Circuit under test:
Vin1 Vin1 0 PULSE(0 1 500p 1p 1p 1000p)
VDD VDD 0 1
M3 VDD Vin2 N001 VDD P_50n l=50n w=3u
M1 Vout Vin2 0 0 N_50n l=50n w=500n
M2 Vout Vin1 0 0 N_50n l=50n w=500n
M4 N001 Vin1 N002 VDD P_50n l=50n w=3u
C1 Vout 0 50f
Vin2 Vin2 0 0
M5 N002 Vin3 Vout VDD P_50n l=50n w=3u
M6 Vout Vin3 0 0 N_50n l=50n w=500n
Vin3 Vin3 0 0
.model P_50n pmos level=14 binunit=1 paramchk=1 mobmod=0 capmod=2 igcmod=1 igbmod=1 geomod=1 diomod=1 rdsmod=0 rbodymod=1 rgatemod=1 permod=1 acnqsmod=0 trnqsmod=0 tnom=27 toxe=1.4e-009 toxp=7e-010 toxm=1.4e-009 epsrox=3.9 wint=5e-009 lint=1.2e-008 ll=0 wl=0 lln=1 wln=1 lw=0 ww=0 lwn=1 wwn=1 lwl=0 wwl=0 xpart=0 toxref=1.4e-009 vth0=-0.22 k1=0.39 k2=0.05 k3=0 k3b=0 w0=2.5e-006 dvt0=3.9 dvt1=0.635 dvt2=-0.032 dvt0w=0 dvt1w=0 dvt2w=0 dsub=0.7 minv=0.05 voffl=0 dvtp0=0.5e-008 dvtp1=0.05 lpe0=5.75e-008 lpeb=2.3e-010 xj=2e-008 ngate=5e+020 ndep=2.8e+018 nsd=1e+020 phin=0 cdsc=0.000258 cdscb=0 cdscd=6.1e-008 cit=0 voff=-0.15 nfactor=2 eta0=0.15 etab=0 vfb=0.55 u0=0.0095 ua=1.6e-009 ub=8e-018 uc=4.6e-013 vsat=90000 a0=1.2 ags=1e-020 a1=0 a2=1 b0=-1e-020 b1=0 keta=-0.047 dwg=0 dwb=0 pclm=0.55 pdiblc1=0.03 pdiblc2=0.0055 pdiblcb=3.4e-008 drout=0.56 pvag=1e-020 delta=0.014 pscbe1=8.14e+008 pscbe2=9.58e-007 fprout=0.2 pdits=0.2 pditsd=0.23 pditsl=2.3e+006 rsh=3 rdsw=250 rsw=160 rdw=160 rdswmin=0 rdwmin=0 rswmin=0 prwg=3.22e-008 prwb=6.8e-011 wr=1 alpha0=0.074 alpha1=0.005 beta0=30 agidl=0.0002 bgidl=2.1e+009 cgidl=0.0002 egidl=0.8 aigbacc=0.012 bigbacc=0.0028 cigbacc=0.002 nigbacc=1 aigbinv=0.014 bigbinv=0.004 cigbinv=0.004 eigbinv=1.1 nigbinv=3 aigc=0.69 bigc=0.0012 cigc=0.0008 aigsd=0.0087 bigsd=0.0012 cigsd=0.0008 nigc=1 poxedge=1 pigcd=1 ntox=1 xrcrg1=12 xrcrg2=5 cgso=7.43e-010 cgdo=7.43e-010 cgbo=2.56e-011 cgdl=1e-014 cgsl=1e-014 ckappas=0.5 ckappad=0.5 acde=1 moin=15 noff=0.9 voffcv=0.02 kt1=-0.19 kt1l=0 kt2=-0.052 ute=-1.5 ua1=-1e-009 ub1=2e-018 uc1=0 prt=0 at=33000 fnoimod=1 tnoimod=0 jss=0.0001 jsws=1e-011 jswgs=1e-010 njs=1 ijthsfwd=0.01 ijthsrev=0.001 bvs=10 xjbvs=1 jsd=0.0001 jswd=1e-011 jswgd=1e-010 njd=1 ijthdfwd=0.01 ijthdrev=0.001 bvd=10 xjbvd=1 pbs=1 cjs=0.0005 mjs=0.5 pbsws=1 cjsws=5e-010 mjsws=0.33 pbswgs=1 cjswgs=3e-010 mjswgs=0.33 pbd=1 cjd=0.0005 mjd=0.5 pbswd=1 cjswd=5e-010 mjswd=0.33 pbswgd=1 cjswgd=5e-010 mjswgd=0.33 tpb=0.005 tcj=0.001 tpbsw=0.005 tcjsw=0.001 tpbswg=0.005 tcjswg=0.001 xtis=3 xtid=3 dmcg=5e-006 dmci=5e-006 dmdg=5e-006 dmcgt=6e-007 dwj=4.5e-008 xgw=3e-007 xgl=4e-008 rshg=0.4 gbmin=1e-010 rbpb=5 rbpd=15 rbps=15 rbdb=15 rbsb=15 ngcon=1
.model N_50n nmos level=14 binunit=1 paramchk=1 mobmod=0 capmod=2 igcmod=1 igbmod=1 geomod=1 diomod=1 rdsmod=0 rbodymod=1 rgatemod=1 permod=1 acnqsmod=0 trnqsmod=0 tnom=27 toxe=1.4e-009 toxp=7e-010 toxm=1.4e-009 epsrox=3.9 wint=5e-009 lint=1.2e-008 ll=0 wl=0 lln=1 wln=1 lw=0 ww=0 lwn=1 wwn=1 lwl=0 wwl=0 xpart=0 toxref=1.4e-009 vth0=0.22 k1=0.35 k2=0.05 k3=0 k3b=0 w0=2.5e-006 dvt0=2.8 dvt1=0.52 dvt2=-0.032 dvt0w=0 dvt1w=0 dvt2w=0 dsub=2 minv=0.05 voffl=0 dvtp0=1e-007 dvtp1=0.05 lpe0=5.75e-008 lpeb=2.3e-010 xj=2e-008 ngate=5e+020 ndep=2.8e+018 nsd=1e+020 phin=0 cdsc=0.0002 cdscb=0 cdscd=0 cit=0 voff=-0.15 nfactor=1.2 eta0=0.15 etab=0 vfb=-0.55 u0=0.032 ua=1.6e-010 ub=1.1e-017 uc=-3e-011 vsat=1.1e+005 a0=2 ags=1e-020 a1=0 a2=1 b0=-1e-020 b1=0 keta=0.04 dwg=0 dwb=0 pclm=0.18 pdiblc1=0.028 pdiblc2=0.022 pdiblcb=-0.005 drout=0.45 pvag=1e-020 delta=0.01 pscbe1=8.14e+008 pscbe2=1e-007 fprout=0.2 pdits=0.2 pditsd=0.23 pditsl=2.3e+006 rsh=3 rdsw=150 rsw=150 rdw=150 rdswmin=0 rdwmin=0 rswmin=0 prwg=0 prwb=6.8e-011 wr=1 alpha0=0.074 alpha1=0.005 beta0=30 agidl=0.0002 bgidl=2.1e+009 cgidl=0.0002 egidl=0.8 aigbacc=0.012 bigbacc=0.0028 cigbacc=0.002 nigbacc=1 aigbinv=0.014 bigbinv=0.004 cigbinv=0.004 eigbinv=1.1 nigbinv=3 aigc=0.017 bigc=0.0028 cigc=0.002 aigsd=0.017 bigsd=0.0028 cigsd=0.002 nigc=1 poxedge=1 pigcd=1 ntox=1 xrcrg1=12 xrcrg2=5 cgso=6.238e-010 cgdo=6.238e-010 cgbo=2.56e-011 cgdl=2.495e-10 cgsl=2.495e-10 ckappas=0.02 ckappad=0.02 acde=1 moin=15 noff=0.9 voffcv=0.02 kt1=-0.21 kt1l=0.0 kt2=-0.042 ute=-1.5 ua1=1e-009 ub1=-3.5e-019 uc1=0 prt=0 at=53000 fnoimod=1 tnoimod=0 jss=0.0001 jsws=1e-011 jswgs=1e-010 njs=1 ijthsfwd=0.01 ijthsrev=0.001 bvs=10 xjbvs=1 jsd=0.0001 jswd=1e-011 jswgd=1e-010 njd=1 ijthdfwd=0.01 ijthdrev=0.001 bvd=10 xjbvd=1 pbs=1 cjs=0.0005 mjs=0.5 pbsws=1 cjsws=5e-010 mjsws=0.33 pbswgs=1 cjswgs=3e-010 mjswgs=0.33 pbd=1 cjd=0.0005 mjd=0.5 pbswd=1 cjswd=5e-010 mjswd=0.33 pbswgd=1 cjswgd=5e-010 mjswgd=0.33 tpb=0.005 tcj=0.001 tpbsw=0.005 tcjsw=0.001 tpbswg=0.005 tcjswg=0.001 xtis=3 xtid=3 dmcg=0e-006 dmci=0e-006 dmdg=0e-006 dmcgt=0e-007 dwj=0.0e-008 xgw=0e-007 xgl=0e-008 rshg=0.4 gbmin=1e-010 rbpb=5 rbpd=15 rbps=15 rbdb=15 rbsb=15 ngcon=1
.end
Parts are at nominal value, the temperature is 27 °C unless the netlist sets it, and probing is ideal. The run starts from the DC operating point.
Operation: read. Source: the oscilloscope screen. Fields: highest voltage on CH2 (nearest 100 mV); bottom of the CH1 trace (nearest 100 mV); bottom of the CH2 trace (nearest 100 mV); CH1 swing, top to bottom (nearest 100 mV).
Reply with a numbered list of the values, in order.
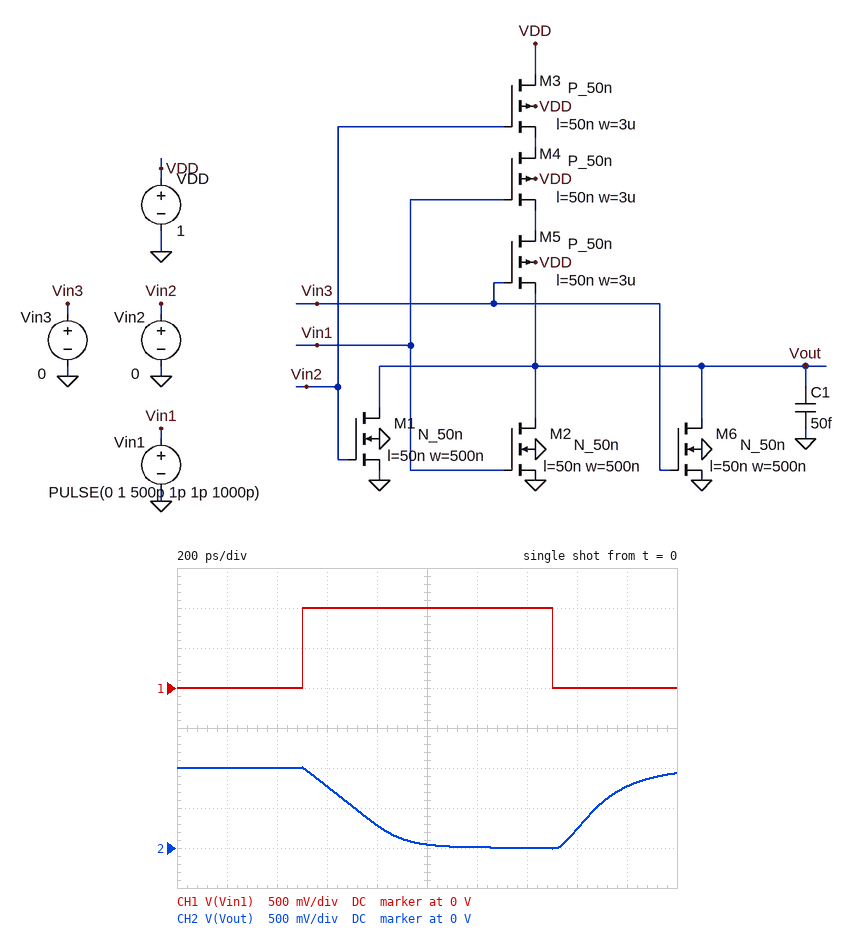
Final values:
1. 1.0 V
2. 0 V
3. 0 V
4. 1.0 V
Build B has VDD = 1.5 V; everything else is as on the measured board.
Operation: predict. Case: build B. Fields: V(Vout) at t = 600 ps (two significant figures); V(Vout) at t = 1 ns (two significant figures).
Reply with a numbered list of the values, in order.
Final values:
1. 1.3 V
2. 520 mV
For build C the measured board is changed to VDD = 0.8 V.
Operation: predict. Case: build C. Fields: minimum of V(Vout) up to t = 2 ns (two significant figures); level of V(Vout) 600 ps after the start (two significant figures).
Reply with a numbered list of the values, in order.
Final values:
1. -6.5 mV
2. 580 mV
